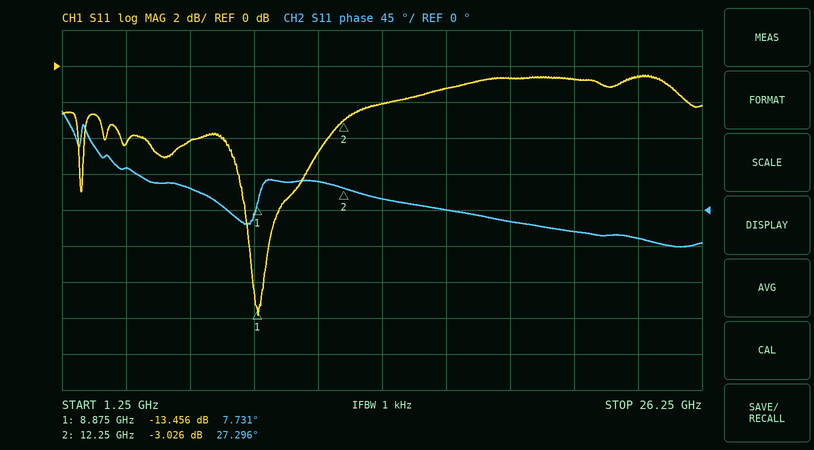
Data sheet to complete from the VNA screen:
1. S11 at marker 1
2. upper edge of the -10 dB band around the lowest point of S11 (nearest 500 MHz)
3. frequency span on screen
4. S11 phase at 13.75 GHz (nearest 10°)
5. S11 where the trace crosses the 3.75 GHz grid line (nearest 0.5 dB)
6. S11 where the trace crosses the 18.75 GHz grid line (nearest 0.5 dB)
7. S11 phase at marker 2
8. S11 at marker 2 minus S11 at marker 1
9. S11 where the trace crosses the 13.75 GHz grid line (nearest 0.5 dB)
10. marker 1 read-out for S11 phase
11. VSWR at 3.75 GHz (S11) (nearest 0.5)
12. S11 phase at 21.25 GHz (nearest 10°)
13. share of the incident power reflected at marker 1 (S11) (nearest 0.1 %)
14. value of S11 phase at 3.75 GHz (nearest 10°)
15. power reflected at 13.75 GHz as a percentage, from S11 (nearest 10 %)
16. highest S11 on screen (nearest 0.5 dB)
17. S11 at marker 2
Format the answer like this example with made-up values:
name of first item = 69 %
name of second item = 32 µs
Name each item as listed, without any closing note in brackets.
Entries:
S11 at marker 1 = -13.456 dB
upper edge of the -10 dB band around the lowest point of S11 = 9.5 GHz
frequency span on screen = 25 GHz
S11 phase at 13.75 GHz = 10°
S11 where the trace crosses the 3.75 GHz grid line = -4.5 dB
S11 where the trace crosses the 18.75 GHz grid line = -0.5 dB
S11 phase at marker 2 = 27.296°
S11 at marker 2 minus S11 at marker 1 = 10.430 dB
S11 where the trace crosses the 13.75 GHz grid line = -2.0 dB
marker 1 read-out for S11 phase = 7.731°
VSWR at 3.75 GHz (S11) = 4.0
S11 phase at 21.25 GHz = -30°
share of the incident power reflected at marker 1 (S11) = 4.5 %
value of S11 phase at 3.75 GHz = 50°
power reflected at 13.75 GHz as a percentage, from S11 = 60 %
highest S11 on screen = -0.5 dB
S11 at marker 2 = -3.026 dB
